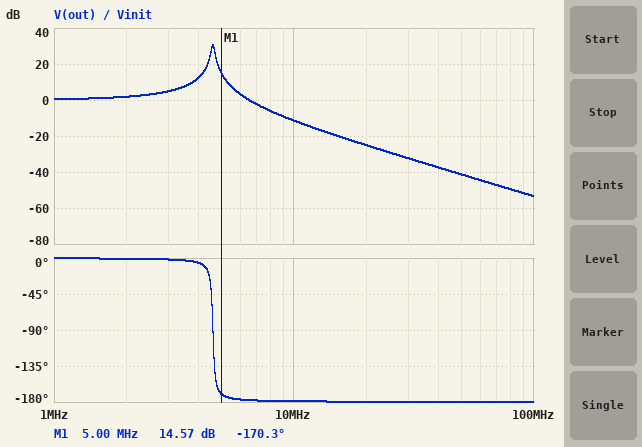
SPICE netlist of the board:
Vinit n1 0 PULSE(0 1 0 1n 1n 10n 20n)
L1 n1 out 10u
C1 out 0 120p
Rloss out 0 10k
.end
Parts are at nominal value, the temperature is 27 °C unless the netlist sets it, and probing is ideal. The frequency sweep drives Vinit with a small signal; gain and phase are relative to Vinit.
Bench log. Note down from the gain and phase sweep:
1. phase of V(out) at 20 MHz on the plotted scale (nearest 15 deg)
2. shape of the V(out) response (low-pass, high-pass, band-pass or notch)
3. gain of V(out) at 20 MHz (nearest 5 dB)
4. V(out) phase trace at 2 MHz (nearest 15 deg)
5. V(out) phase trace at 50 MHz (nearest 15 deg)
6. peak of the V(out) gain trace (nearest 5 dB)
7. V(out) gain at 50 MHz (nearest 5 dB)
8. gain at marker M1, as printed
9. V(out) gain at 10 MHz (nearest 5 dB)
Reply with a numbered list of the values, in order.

1. -180 deg
2. low-pass
3. -25 dB
4. 0 deg
5. -180 deg
6. 30 dB
7. -40 dB
8. 14.57 dB
9. -10 dB
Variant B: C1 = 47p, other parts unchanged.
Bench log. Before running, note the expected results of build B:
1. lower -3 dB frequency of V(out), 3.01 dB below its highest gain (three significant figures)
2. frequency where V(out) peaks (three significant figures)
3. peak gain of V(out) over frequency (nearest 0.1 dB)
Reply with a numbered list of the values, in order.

1. 7.17 MHz
2. 7.34 MHz
3. 26.7 dB
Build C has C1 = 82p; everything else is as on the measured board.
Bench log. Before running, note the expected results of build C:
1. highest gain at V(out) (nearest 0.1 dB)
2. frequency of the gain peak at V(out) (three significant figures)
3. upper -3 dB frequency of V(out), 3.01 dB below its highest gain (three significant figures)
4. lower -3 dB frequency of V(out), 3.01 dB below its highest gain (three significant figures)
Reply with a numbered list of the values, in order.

1. 29.1 dB
2. 5.56 MHz
3. 5.65 MHz
4. 5.46 MHz
